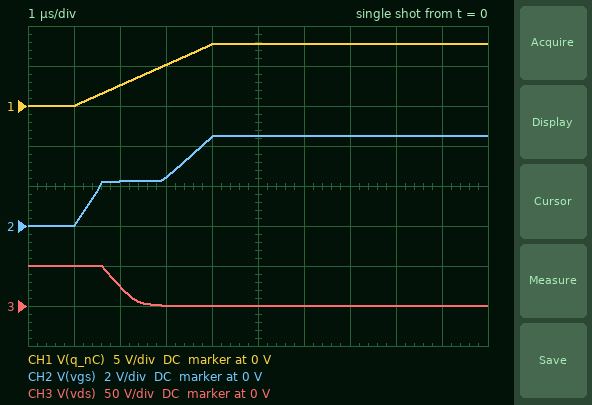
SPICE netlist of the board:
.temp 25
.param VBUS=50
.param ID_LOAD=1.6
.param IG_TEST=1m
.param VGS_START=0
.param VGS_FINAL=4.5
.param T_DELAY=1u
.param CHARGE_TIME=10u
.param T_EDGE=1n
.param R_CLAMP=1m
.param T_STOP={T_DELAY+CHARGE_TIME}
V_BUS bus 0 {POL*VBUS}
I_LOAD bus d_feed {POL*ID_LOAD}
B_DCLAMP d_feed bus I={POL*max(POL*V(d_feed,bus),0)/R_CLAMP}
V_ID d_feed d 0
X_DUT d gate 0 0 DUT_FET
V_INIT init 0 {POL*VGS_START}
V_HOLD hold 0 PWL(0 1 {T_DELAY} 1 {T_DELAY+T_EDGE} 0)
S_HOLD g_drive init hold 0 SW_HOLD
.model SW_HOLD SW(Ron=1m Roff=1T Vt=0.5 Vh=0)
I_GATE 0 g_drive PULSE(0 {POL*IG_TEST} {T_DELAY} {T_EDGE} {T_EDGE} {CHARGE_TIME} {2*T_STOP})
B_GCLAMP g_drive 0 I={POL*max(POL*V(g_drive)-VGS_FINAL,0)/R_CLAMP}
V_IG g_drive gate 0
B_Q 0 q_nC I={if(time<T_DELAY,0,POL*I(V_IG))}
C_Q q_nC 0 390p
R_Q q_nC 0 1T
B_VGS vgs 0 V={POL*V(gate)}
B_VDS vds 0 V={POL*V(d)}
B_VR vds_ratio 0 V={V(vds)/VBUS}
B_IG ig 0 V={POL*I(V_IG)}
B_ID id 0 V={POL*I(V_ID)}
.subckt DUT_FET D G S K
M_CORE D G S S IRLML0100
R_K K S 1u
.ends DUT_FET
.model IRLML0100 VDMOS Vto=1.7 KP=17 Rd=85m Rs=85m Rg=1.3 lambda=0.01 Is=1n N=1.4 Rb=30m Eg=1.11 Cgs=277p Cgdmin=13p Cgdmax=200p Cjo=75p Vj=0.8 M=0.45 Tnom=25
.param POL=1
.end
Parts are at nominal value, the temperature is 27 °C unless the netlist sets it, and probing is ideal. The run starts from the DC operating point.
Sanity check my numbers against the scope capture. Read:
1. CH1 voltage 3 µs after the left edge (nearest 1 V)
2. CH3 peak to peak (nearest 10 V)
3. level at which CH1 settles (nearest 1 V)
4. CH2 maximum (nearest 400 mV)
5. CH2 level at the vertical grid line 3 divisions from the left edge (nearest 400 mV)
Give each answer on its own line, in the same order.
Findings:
5 V
50 V
8 V
4.4 V
2.4 V
